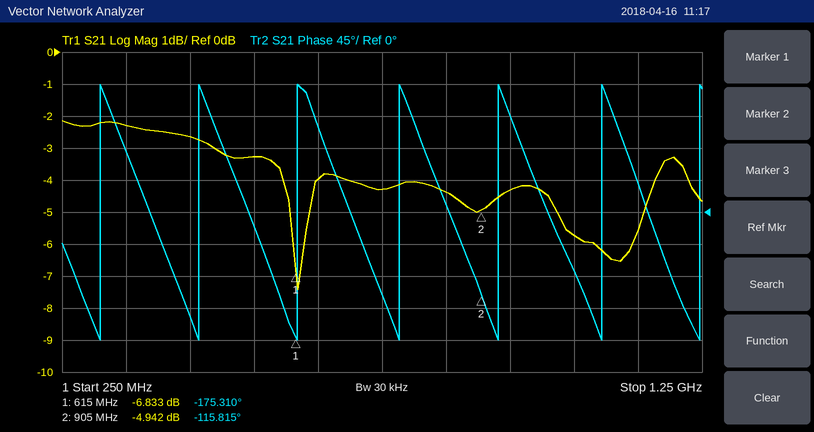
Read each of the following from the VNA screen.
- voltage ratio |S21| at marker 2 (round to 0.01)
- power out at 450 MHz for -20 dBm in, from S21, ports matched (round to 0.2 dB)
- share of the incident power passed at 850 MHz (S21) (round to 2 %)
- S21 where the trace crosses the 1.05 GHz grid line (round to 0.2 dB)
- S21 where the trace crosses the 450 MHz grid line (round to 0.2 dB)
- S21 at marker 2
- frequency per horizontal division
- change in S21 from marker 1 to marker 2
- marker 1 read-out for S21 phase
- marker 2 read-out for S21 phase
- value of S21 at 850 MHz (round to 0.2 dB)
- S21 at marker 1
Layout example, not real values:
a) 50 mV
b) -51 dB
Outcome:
a) 0.57
b) -22.6 dBm
c) 36 %
d) -5.8 dB
e) -2.6 dB
f) -4.942 dB
g) 100 MHz
h) 1.891 dB
i) -175.310°
j) -115.815°
k) -4.4 dB
l) -6.833 dB
